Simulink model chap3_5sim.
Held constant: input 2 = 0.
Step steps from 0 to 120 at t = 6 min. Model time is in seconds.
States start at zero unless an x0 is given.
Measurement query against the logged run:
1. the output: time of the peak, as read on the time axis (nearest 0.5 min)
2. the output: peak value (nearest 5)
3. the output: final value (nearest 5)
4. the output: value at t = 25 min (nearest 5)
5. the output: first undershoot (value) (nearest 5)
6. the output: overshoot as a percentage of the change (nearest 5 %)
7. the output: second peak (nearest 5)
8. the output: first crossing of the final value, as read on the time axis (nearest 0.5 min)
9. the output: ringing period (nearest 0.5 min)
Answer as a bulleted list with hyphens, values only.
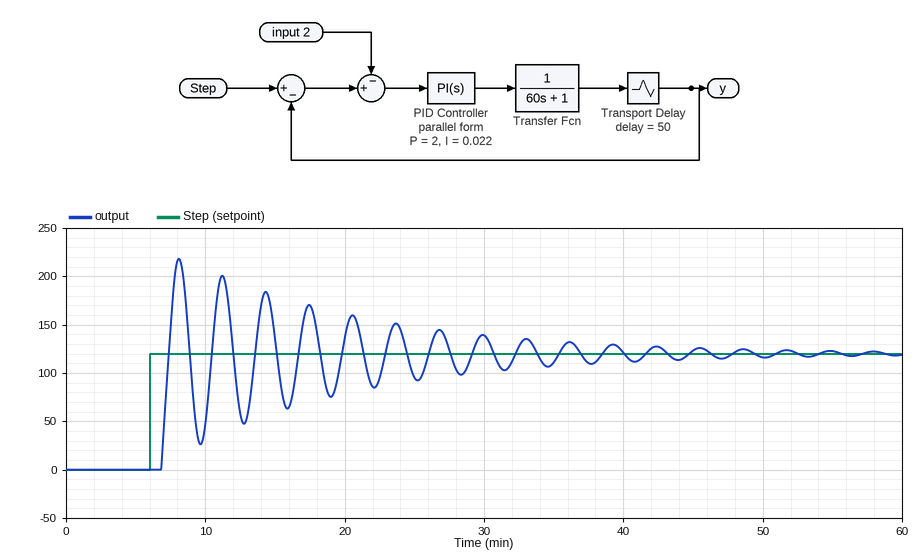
- 8.0 min
- 220
- 120
- 95
- 25
- 80 %
- 200
- 7.5 min
- 3.0 min
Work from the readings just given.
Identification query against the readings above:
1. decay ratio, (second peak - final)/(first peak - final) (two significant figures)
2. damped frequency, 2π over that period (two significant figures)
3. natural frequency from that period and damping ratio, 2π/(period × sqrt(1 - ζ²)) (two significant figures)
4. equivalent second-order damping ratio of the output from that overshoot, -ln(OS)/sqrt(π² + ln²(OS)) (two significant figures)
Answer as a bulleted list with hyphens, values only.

- 0.80
- 2.1 rad/min
- 2.1 rad/min
- 0.071
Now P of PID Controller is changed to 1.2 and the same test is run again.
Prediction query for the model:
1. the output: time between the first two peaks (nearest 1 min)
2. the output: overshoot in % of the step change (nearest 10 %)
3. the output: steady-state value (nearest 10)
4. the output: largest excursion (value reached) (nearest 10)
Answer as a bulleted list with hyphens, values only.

- 4 min
- 60 %
- 120
- 190
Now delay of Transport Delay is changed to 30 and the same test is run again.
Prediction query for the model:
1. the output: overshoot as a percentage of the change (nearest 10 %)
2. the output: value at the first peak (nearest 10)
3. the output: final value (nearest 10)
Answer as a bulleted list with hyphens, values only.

- 30 %
- 160
- 120
